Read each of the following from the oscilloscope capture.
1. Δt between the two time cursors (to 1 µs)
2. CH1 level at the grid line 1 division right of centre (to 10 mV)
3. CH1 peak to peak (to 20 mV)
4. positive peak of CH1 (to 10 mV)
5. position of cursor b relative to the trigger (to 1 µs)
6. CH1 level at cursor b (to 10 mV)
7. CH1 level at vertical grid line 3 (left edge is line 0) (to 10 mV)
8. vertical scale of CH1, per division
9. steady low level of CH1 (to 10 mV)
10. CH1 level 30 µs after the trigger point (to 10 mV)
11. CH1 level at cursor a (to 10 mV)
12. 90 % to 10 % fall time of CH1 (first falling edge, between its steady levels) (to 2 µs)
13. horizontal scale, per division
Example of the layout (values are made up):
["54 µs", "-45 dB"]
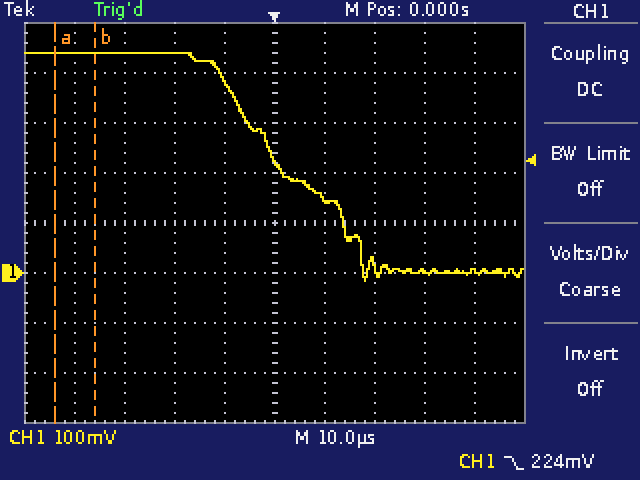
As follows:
["8 µs", "150 mV", "460 mV", "440 mV", "-36 µs", "440 mV", "440 mV", "100 mV", "0 mV", "0 mV", "440 mV", "28 µs", "10 µs"]
